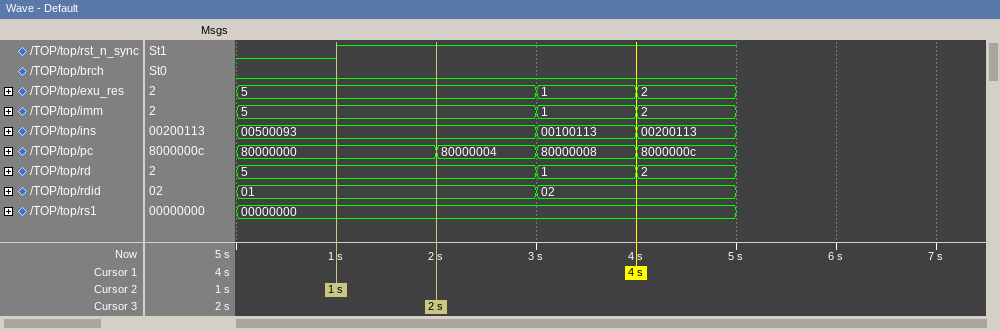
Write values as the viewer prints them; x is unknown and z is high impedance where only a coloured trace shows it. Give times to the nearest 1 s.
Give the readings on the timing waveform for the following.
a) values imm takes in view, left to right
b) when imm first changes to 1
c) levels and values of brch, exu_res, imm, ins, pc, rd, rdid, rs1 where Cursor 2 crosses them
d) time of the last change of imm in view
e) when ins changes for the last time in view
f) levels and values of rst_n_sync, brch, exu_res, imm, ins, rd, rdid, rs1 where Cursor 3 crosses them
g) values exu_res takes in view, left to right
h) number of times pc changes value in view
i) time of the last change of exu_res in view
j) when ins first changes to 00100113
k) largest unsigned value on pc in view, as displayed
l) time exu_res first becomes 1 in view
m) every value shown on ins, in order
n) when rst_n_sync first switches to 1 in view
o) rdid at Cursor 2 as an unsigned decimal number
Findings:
5, 1, 2
3 s
brch=0, exu_res=5, imm=5, ins=00500093, pc=80000000, rd=5, rdid=01, rs1=00000000
4 s
4 s
rst_n_sync=1, brch=0, exu_res=5, imm=5, ins=00500093, rd=5, rdid=01, rs1=00000000
5, 1, 2
3
4 s
3 s
8000000c
3 s
00500093, 00100113, 00200113
1 s
1
